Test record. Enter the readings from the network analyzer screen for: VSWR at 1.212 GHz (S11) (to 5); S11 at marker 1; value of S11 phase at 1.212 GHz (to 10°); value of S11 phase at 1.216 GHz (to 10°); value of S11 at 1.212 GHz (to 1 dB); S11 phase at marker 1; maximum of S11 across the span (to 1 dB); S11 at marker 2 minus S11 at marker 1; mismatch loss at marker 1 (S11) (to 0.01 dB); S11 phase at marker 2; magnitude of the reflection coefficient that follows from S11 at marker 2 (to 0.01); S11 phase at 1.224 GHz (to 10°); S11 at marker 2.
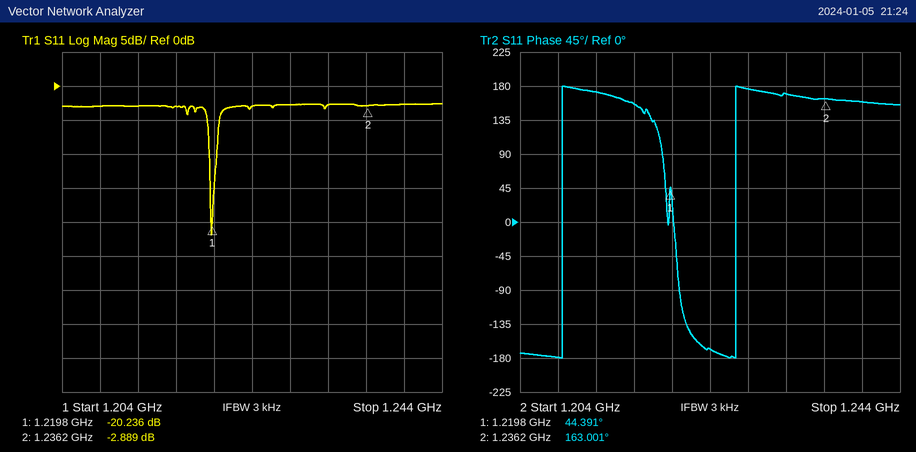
5
-20.236 dB
170°
160°
-3 dB
44.391°
-3 dB
17.347 dB
0.04 dB
163.001°
0.72
-170°
-2.889 dB
